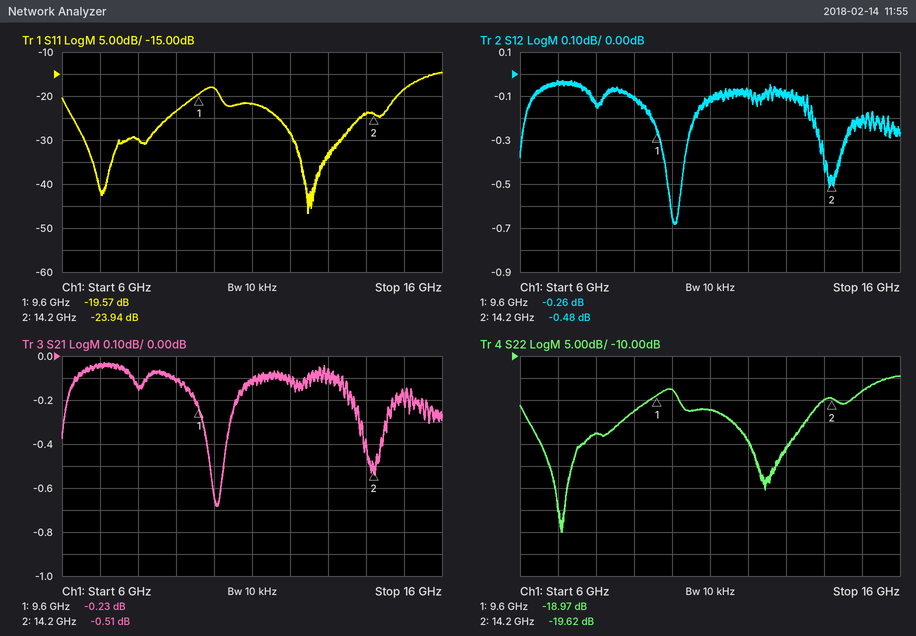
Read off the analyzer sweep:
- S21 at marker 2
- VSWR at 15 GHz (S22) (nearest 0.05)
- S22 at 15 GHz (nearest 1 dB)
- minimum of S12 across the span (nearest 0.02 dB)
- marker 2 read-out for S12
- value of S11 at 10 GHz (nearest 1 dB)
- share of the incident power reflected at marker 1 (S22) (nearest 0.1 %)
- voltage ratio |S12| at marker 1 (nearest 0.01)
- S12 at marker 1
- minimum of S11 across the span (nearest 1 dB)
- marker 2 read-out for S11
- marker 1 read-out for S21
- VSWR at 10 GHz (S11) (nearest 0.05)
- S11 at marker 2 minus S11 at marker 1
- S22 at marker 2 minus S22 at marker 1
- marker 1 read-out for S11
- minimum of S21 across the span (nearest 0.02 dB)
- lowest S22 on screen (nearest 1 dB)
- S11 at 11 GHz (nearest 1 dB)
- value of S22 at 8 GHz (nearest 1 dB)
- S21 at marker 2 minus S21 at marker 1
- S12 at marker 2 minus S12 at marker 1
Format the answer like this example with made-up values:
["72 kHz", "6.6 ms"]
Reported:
["-0.51 dB", "1.30", "-18 dB", "-0.68 dB", "-0.48 dB", "-18 dB", "1.3 %", "0.97", "-0.26 dB", "-47 dB", "-23.94 dB", "-0.23 dB", "1.30", "-4.37 dB", "-0.65 dB", "-19.57 dB", "-0.68 dB", "-50 dB", "-22 dB", "-28 dB", "-0.28 dB", "-0.22 dB"]
